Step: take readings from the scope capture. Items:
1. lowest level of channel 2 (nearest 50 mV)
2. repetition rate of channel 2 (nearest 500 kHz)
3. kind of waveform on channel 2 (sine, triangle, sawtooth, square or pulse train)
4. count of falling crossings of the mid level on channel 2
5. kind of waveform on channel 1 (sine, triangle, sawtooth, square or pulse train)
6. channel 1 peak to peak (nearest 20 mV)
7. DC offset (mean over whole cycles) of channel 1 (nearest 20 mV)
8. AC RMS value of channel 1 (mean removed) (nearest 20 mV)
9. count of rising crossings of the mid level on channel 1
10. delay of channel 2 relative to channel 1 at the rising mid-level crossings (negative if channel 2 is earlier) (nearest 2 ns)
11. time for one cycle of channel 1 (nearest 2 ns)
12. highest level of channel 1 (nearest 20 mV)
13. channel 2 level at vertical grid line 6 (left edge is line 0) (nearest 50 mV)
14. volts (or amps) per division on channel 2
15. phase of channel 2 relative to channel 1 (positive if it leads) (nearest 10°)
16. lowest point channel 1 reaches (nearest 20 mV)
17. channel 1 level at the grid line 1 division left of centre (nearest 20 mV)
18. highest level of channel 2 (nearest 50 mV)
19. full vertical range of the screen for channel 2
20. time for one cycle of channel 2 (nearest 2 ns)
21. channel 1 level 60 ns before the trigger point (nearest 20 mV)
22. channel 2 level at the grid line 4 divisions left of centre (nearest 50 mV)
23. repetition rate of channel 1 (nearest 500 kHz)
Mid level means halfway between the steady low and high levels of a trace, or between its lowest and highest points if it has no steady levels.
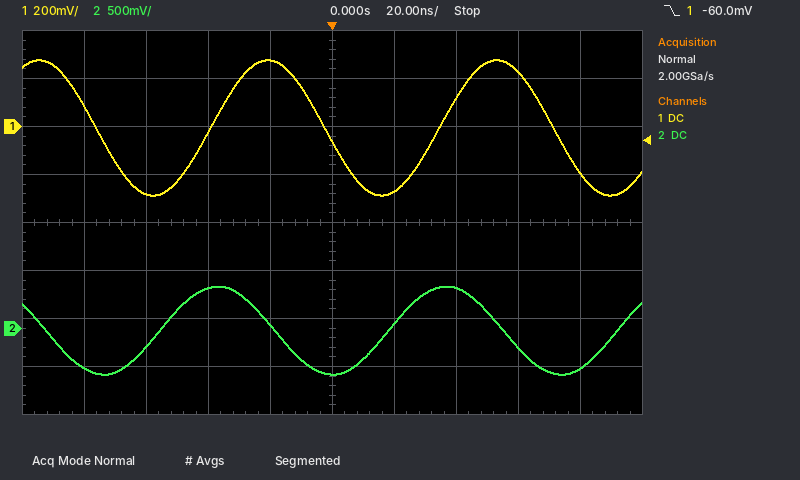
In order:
-500 mV
13.5 MHz
sine
3
sine
560 mV
0 mV
200 mV
2
-16 ns
74 ns
280 mV
50 mV
500 mV
+80°
-280 mV
280 mV
450 mV
4 V
74 ns
-280 mV
-400 mV
13.5 MHz
